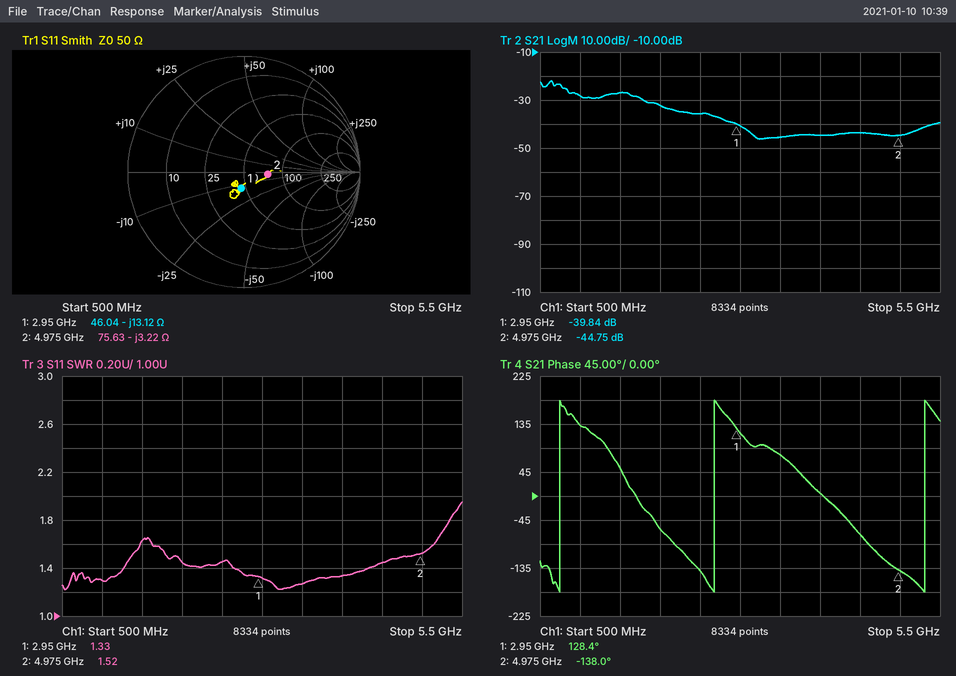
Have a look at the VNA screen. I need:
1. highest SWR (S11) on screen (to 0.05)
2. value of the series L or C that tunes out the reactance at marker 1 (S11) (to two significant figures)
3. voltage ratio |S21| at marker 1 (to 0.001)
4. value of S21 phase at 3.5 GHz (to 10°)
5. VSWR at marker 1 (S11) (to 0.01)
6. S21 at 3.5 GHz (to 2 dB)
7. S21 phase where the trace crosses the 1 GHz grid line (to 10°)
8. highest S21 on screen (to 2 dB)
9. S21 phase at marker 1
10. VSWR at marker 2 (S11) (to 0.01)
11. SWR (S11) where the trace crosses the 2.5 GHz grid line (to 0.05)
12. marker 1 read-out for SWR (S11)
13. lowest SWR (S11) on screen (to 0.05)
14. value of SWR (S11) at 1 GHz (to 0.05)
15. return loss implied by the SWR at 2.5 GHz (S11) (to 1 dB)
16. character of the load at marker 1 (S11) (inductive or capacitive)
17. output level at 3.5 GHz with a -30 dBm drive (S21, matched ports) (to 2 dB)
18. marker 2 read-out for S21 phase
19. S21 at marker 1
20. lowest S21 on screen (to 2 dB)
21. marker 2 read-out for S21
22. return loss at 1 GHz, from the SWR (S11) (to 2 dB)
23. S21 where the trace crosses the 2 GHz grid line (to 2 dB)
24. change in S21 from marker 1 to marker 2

1.95
710 pH
0.010
80°
1.33
-46 dB
130°
-22 dB
128.4°
1.52
1.45
1.33
1.20
1.30
15 dB
capacitive
-76 dBm
-138.0°
-39.84 dB
-46 dB
-44.75 dB
18 dB
-32 dB
-4.91 dB
